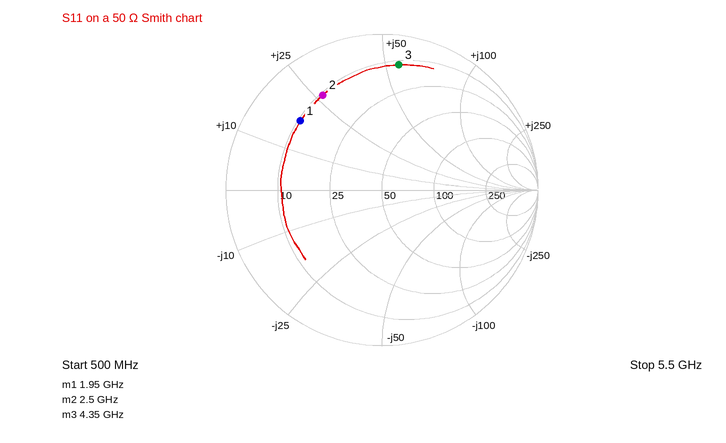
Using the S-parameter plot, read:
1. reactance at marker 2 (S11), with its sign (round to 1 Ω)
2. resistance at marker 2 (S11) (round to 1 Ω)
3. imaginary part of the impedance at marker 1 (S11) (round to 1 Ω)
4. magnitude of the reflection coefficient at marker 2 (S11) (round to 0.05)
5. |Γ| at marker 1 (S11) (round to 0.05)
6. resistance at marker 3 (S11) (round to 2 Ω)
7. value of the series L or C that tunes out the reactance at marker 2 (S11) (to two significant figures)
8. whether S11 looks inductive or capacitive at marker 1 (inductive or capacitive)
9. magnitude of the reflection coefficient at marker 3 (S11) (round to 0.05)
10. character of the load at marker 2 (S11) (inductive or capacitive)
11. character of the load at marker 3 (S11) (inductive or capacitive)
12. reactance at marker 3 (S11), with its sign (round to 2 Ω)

+27 Ω
11 Ω
+18 Ω
0.70
0.70
12 Ω
2.4 pF
inductive
0.80
inductive
inductive
+56 Ω
